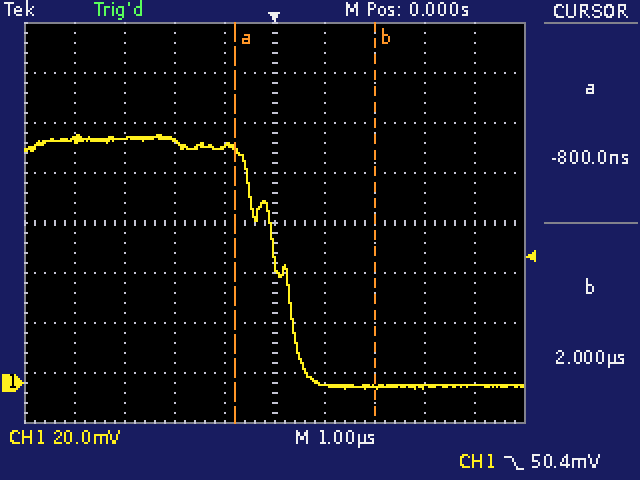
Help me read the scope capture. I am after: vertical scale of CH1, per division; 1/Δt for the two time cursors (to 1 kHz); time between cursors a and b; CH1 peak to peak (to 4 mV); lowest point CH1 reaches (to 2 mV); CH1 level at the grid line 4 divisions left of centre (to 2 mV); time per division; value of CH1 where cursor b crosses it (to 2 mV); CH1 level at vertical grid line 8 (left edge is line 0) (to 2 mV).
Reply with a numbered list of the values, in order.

1. 20 mV
2. 357 kHz
3. 2.8 µs
4. 100 mV
5. -2 mV
6. 98 mV
7. 1 µs
8. -2 mV
9. -2 mV
